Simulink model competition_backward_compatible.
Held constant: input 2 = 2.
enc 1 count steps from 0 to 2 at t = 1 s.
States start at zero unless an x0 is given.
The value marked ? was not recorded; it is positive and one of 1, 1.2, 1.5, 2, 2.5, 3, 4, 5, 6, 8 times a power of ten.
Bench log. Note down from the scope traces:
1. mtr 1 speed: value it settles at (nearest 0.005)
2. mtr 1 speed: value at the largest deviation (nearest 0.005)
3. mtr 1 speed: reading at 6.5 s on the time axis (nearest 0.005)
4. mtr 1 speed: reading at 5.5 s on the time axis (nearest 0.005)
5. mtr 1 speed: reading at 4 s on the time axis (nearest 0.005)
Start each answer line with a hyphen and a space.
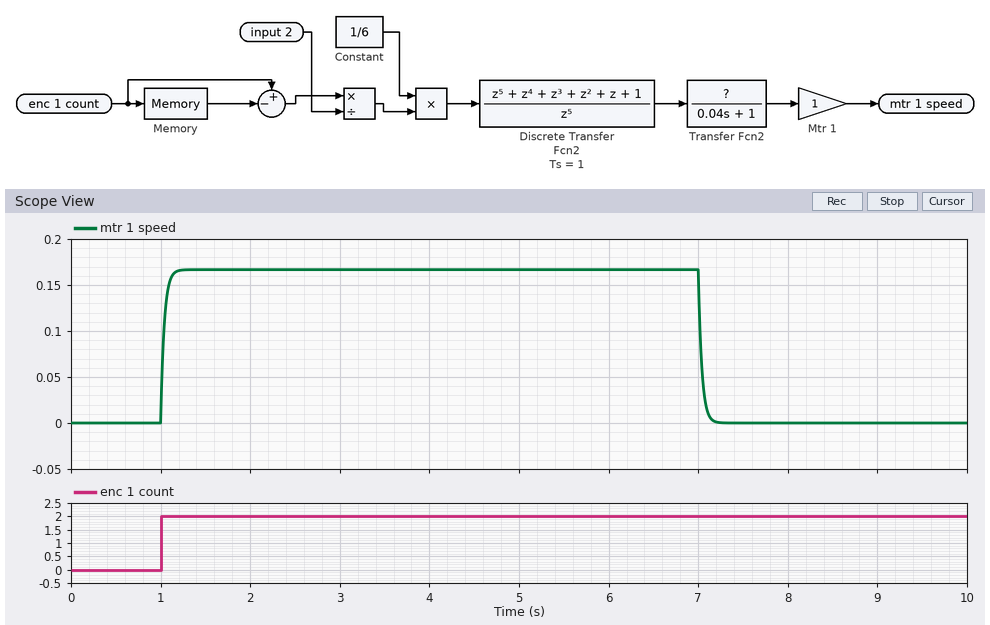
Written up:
- 0.000
- 0.165
- 0.165
- 0.165
- 0.165
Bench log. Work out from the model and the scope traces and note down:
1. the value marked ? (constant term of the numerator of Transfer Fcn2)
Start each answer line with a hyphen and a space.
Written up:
- 1
